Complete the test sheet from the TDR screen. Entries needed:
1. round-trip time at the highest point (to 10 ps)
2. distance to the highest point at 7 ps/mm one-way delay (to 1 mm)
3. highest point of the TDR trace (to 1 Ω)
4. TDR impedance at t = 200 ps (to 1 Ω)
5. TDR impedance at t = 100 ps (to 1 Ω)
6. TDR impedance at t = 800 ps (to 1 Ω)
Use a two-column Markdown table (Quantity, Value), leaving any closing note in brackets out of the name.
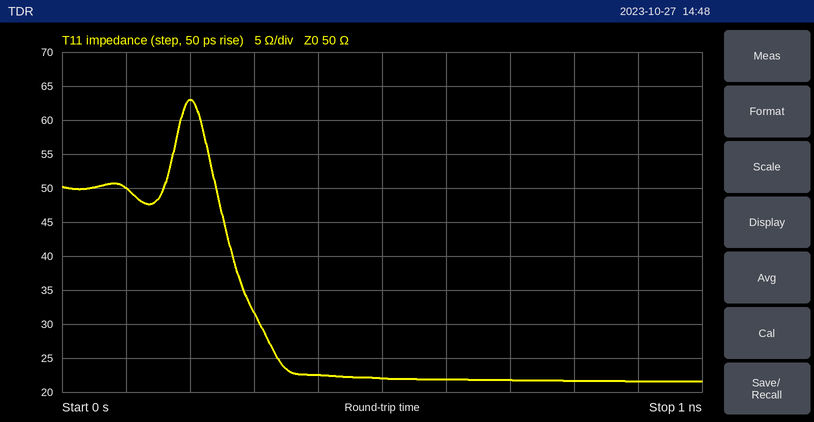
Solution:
| Quantity | Value |
|---|---|
| round-trip time at the highest point | 200 ps |
| distance to the highest point at 7 ps/mm one-way delay | 14 mm |
| highest point of the TDR trace | 63 Ω |
| TDR impedance at t = 200 ps | 63 Ω |
| TDR impedance at t = 100 ps | 50 Ω |
| TDR impedance at t = 800 ps | 22 Ω |
